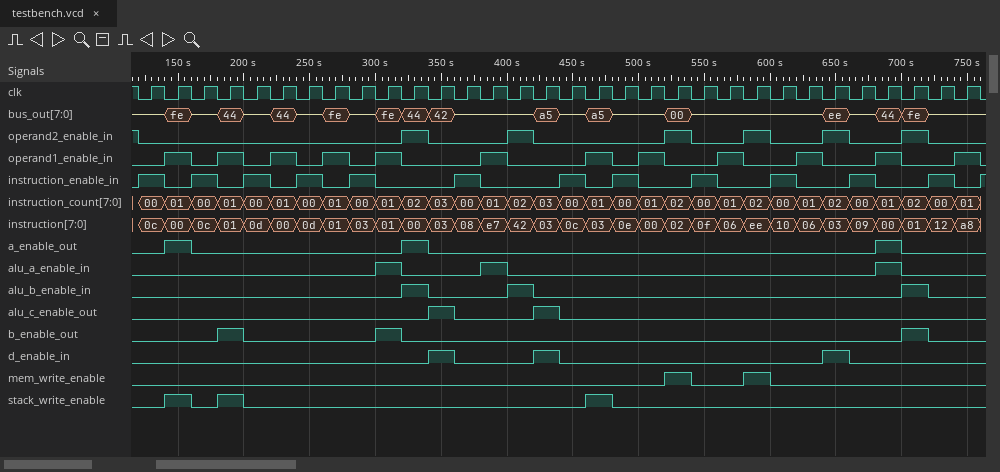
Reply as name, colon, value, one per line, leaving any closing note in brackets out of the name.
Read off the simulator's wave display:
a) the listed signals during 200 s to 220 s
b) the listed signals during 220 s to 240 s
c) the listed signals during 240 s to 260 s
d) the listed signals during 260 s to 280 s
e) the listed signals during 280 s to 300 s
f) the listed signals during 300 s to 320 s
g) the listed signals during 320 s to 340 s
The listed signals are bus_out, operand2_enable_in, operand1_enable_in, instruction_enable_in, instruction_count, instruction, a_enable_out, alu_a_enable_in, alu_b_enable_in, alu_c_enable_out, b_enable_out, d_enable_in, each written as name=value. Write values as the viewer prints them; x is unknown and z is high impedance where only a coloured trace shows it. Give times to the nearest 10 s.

the listed signals during 200 s to 220 s: bus_out=z, operand2_enable_in=0, operand1_enable_in=0, instruction_enable_in=1, instruction_count=00, instruction=0d, a_enable_out=0, alu_a_enable_in=0, alu_b_enable_in=0, alu_c_enable_out=0, b_enable_out=0, d_enable_in=0
the listed signals during 220 s to 240 s: bus_out=44, operand2_enable_in=0, operand1_enable_in=1, instruction_enable_in=0, instruction_count=01, instruction=00, a_enable_out=0, alu_a_enable_in=0, alu_b_enable_in=0, alu_c_enable_out=0, b_enable_out=0, d_enable_in=0
the listed signals during 240 s to 260 s: bus_out=z, operand2_enable_in=0, operand1_enable_in=0, instruction_enable_in=1, instruction_count=00, instruction=0d, a_enable_out=0, alu_a_enable_in=0, alu_b_enable_in=0, alu_c_enable_out=0, b_enable_out=0, d_enable_in=0
the listed signals during 260 s to 280 s: bus_out=fe, operand2_enable_in=0, operand1_enable_in=1, instruction_enable_in=0, instruction_count=01, instruction=01, a_enable_out=0, alu_a_enable_in=0, alu_b_enable_in=0, alu_c_enable_out=0, b_enable_out=0, d_enable_in=0
the listed signals during 280 s to 300 s: bus_out=z, operand2_enable_in=0, operand1_enable_in=0, instruction_enable_in=1, instruction_count=00, instruction=03, a_enable_out=0, alu_a_enable_in=0, alu_b_enable_in=0, alu_c_enable_out=0, b_enable_out=0, d_enable_in=0
the listed signals during 300 s to 320 s: bus_out=fe, operand2_enable_in=0, operand1_enable_in=1, instruction_enable_in=0, instruction_count=01, instruction=01, a_enable_out=0, alu_a_enable_in=1, alu_b_enable_in=0, alu_c_enable_out=0, b_enable_out=1, d_enable_in=0
the listed signals during 320 s to 340 s: bus_out=44, operand2_enable_in=1, operand1_enable_in=0, instruction_enable_in=0, instruction_count=02, instruction=00, a_enable_out=1, alu_a_enable_in=0, alu_b_enable_in=1, alu_c_enable_out=0, b_enable_out=0, d_enable_in=0
